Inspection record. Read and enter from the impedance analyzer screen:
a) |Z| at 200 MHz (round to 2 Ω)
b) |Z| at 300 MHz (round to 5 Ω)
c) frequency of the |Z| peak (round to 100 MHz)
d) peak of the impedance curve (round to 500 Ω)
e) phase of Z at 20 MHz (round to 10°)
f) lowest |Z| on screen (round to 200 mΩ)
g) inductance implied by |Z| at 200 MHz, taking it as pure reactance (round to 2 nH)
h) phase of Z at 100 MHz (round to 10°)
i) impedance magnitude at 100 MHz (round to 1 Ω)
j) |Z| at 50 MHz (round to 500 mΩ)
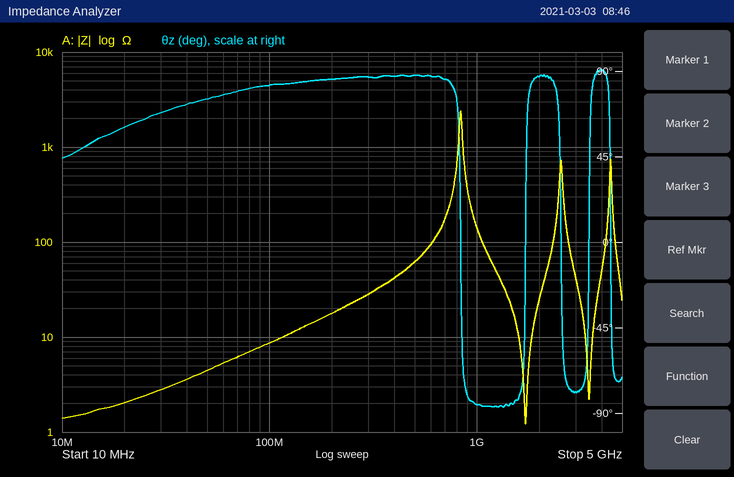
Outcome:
18 Ω
30 Ω
800 MHz
2.5 kΩ
60°
1.2 Ω
14 nH
80°
9 Ω
4.5 Ω
